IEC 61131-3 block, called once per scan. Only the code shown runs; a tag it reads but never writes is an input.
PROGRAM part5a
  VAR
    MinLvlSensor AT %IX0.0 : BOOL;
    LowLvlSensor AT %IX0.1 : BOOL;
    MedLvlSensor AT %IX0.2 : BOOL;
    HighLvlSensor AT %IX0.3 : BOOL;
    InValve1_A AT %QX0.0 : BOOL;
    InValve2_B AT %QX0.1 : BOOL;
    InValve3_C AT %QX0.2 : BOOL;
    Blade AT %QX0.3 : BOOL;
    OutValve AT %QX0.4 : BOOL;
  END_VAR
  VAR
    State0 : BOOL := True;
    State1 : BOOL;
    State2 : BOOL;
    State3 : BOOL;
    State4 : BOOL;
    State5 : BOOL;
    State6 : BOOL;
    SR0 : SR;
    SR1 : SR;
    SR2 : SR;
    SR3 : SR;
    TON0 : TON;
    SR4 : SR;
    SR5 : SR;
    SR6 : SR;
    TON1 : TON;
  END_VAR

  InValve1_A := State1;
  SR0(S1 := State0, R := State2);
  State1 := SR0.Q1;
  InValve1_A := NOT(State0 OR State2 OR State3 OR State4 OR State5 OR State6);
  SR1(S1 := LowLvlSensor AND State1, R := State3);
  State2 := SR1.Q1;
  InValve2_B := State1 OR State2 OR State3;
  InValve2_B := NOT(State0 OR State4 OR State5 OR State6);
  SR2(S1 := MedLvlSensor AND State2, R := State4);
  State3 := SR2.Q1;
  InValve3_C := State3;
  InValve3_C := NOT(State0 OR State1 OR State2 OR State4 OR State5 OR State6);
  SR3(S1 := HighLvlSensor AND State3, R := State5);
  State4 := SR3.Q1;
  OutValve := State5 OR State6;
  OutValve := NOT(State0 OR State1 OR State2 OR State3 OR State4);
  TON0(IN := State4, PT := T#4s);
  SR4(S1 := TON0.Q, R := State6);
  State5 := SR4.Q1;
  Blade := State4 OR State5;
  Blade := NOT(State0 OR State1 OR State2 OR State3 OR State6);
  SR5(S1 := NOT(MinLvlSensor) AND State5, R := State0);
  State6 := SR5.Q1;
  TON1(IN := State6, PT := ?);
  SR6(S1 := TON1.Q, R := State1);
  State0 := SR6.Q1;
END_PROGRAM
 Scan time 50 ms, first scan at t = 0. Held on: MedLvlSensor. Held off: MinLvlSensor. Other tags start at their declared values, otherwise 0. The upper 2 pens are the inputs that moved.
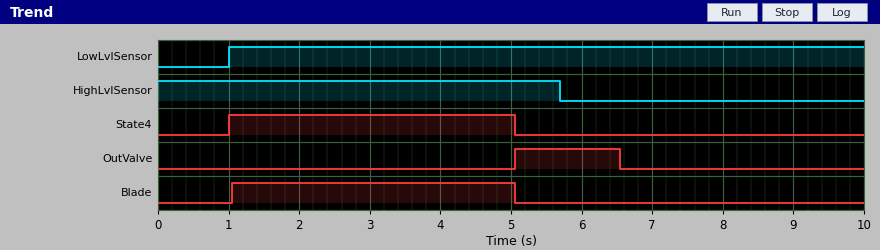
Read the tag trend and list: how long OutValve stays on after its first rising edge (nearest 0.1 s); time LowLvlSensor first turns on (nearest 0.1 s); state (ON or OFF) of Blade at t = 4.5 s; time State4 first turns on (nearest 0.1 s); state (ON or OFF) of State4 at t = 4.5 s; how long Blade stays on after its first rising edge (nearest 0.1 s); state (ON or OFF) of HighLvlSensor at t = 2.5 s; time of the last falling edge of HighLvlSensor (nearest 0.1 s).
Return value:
1.5 s
1.0 s
ON
1.0 s
ON
4.0 s
ON
5.7 s
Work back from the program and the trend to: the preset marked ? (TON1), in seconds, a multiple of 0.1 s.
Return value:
1.5 s
